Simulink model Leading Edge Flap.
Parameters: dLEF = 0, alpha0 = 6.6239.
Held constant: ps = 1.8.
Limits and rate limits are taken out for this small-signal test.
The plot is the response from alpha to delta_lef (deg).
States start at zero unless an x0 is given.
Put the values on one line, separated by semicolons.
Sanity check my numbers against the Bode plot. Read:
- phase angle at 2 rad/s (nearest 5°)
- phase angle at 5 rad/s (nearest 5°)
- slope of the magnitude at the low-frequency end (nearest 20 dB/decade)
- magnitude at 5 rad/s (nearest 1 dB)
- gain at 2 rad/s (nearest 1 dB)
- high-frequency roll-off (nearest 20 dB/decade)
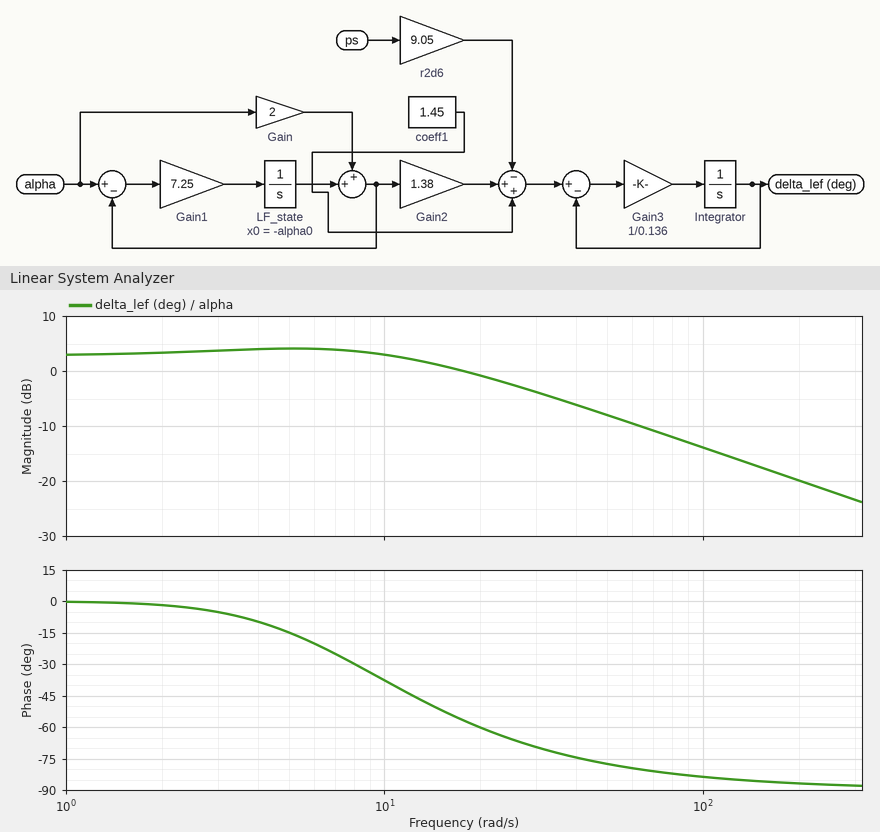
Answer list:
0°; -15°; 0 dB/decade; 4 dB; 3 dB; -20 dB/decade
